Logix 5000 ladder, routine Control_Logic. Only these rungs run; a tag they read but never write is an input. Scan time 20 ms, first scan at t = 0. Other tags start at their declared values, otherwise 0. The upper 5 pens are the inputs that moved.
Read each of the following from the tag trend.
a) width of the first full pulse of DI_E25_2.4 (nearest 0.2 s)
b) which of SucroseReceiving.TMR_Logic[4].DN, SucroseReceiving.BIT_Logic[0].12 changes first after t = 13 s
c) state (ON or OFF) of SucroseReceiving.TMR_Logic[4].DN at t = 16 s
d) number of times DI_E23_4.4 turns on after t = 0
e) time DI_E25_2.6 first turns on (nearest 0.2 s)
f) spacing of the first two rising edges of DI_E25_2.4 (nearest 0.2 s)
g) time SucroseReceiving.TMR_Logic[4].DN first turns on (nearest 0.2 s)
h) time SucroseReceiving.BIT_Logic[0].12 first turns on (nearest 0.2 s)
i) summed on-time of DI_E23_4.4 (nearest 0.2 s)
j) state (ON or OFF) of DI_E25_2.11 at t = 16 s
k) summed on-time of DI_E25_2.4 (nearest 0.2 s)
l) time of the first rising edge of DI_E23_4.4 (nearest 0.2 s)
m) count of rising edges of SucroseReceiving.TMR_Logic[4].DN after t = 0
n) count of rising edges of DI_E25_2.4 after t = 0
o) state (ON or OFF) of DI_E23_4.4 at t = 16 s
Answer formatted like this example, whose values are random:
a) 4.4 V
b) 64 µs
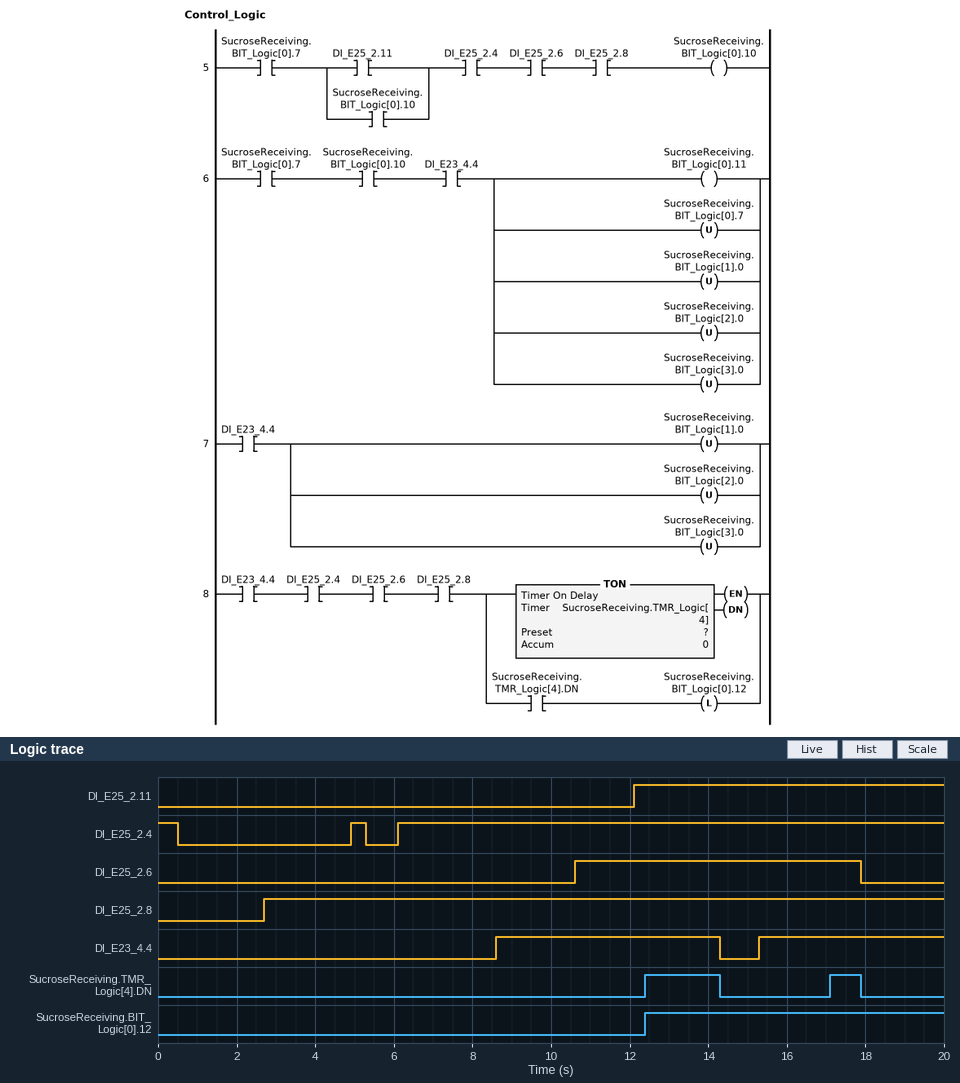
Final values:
a) 0.4 s
b) SucroseReceiving.TMR_Logic[4].DN
c) OFF
d) 2
e) 10.6 s
f) 1.2 s
g) 12.4 s
h) 12.4 s
i) 10.4 s
j) ON
k) 14.8 s
l) 8.6 s
m) 2
n) 2
o) ON
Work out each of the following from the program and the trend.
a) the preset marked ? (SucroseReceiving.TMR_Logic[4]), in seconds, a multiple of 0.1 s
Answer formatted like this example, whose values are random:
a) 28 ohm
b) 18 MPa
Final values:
a) 1.8 s
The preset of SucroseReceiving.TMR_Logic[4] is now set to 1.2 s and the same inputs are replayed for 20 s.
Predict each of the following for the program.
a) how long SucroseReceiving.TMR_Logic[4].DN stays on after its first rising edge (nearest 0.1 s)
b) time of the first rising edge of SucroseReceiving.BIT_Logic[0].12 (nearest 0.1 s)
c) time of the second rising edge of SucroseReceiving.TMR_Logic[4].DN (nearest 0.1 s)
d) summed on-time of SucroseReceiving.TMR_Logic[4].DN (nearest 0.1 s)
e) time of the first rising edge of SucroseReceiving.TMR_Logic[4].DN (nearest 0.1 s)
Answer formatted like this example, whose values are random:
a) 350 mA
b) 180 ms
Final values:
a) 2.5 s
b) 11.8 s
c) 16.5 s
d) 3.9 s
e) 11.8 s
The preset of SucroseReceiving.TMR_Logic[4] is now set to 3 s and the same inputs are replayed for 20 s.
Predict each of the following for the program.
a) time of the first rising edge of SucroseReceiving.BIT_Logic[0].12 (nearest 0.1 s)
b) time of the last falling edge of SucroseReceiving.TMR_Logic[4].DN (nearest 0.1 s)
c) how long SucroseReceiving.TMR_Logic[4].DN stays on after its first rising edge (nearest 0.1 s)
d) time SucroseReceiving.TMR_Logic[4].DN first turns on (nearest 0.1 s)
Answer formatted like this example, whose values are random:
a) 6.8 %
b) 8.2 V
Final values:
a) 13.6 s
b) 14.3 s
c) 0.7 s
d) 13.6 s
